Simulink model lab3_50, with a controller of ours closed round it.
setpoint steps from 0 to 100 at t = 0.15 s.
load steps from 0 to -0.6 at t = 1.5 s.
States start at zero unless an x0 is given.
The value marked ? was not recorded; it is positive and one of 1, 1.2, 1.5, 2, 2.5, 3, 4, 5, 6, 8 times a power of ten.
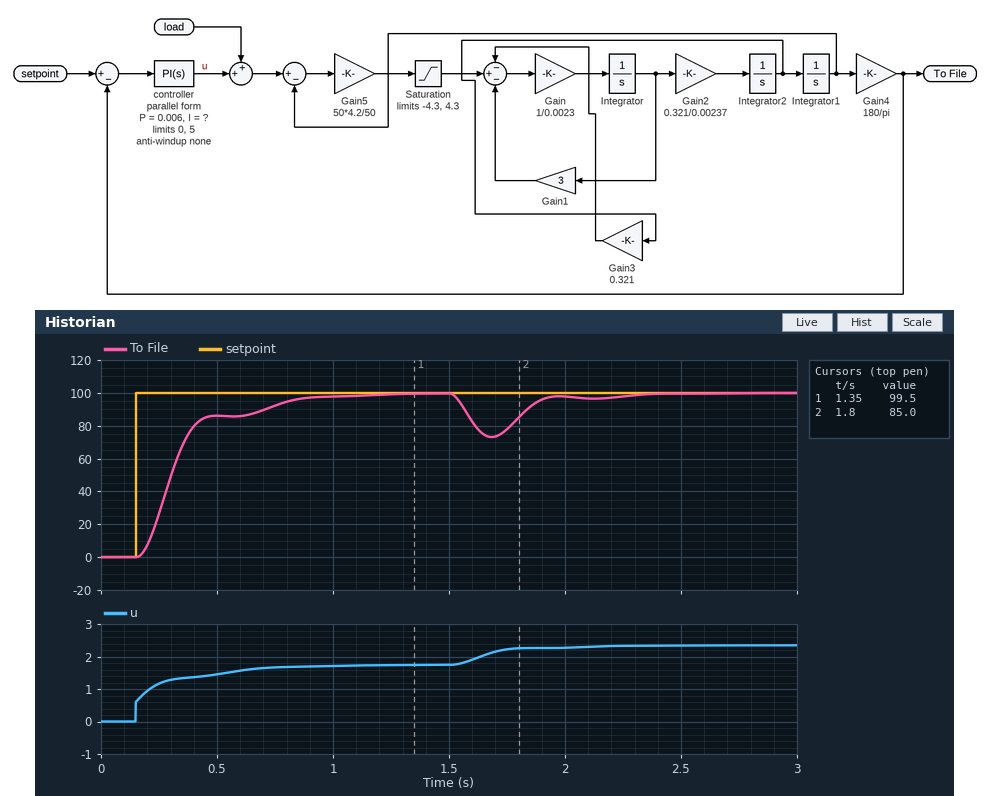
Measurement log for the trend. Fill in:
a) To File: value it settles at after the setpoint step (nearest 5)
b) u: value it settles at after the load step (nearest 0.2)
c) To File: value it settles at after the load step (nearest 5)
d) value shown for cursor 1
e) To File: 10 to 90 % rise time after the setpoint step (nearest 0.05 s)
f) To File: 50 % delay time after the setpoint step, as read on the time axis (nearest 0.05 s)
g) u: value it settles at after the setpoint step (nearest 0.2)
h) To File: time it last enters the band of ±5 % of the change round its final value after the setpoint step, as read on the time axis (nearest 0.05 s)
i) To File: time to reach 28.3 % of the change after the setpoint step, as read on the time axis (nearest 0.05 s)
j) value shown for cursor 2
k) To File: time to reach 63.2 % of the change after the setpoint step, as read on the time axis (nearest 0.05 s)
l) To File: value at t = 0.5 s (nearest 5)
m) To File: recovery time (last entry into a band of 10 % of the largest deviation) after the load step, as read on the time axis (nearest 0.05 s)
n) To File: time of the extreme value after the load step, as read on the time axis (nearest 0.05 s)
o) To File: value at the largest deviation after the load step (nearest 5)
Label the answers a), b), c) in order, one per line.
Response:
a) 100
b) 2.4
c) 100
d) 99.5
e) 0.50 s
f) 0.30 s
g) 1.8
h) 0.80 s
i) 0.25 s
j) 85.0
k) 0.35 s
l) 85
m) 2.20 s
n) 1.70 s
o) 75
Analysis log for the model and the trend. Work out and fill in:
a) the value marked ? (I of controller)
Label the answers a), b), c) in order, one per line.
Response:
a) 0.08
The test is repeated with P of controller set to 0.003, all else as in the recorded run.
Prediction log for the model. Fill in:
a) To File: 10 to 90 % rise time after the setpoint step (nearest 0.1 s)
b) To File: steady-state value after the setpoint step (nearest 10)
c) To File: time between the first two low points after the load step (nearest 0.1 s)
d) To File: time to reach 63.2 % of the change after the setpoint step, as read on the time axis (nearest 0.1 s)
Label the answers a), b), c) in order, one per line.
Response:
a) 0.3 s
b) 100
c) 0.5 s
d) 0.4 s
